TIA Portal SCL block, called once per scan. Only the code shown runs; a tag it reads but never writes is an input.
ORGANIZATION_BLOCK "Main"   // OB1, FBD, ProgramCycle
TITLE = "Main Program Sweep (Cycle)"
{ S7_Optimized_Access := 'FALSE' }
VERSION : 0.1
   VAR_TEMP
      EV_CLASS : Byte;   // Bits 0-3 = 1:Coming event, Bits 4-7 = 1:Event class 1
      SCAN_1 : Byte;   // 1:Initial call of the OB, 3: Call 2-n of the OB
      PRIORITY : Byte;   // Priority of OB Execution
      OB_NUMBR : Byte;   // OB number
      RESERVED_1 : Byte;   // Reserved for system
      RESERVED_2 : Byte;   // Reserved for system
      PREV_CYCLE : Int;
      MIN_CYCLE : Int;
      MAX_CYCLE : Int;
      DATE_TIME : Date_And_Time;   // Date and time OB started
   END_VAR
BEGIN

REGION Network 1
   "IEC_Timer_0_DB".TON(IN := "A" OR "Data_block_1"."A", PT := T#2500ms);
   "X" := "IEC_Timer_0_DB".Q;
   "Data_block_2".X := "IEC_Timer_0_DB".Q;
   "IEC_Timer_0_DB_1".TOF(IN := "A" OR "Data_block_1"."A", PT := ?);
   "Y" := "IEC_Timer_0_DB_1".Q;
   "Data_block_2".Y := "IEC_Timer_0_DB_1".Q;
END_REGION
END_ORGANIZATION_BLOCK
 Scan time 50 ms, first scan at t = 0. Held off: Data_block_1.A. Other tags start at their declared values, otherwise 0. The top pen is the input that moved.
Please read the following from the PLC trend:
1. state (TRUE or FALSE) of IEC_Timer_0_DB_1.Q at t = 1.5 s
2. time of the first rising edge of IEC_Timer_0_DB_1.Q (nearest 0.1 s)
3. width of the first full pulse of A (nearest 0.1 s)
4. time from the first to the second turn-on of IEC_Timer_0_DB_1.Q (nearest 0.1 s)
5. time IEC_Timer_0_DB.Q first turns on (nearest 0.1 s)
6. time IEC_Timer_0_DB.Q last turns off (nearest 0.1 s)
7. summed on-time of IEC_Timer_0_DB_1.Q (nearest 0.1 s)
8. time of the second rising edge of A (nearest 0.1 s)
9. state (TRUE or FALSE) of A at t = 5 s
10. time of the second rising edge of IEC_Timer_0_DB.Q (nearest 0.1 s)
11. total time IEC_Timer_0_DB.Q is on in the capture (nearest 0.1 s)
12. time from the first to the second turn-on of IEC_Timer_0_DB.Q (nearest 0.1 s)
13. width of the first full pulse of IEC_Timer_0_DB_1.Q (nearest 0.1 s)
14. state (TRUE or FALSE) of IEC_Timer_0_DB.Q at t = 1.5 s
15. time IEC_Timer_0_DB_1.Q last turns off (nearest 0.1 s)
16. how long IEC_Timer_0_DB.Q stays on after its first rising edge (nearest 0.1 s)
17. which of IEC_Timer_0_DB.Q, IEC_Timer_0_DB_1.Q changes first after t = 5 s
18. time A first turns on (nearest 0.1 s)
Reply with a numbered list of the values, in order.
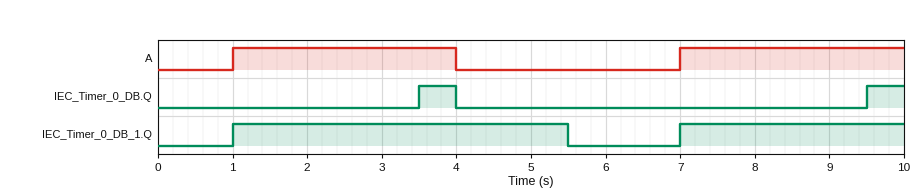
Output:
1. TRUE
2. 1.0 s
3. 3.0 s
4. 6.0 s
5. 3.5 s
6. 4.0 s
7. 7.5 s
8. 7.0 s
9. FALSE
10. 9.5 s
11. 1.0 s
12. 6.0 s
13. 4.5 s
14. FALSE
15. 5.5 s
16. 0.5 s
17. IEC_Timer_0_DB_1.Q
18. 1.0 s
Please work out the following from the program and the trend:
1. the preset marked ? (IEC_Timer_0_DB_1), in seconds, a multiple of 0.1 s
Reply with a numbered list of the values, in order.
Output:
1. 1.5 s
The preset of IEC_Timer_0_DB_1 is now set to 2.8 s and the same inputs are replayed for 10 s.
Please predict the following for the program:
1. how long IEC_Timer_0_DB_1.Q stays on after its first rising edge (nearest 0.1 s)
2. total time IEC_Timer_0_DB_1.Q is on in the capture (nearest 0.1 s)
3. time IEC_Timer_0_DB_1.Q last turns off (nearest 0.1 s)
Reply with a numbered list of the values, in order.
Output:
1. 5.8 s
2. 8.8 s
3. 6.8 s
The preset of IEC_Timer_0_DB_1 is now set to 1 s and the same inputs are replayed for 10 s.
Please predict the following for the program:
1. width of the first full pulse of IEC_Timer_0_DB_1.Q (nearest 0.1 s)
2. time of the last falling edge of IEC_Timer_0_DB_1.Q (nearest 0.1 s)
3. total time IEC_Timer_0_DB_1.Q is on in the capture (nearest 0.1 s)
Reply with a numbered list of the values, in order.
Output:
1. 4.0 s
2. 5.0 s
3. 7.0 s
